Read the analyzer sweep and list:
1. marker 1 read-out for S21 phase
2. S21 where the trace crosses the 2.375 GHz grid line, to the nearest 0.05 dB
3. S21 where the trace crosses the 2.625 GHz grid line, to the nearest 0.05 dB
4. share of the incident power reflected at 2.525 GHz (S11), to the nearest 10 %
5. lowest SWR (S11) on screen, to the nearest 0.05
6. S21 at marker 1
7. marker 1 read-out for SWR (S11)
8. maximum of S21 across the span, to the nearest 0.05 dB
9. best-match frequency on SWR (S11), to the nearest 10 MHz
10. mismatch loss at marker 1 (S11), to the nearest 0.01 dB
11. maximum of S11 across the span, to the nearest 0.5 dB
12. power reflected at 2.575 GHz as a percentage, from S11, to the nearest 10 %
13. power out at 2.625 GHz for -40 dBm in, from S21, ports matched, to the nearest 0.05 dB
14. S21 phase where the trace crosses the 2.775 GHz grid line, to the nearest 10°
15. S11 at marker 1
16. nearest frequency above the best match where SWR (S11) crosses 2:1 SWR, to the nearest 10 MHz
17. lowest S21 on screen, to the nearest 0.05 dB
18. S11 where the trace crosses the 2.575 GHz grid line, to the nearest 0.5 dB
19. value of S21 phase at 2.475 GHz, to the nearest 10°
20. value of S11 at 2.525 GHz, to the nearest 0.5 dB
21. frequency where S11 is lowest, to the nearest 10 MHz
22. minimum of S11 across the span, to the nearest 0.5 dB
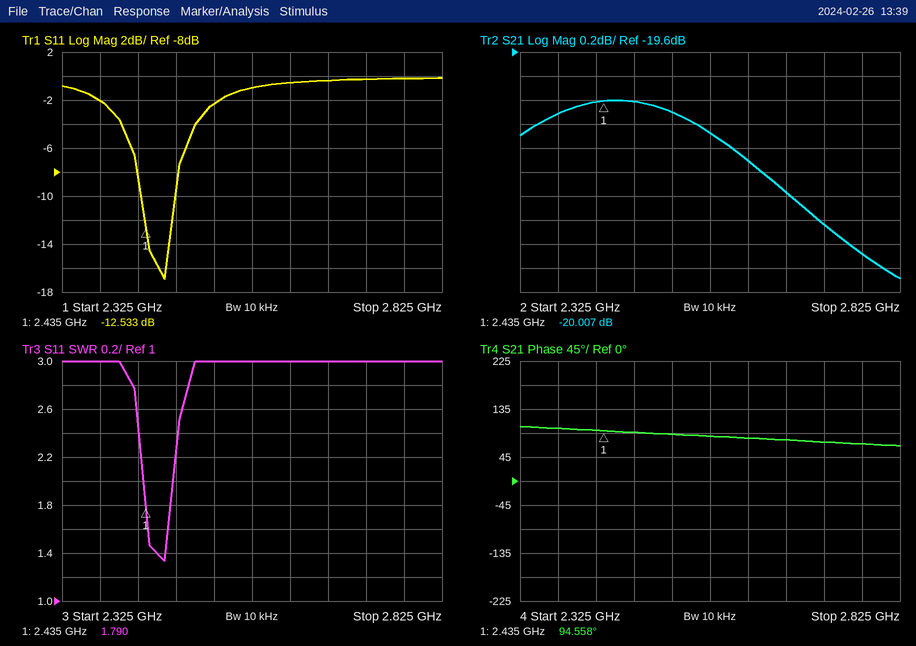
94.558°
-20.10 dB
-20.50 dB
60 %
1.35
-20.007 dB
1.790
-20.00 dB
2.46 GHz
0.25 dB
0.0 dB
80 %
-60.50 dBm
70°
-12.533 dB
2.47 GHz
-21.50 dB
-1.0 dB
90°
-2.5 dB
2.46 GHz
-17.0 dB
